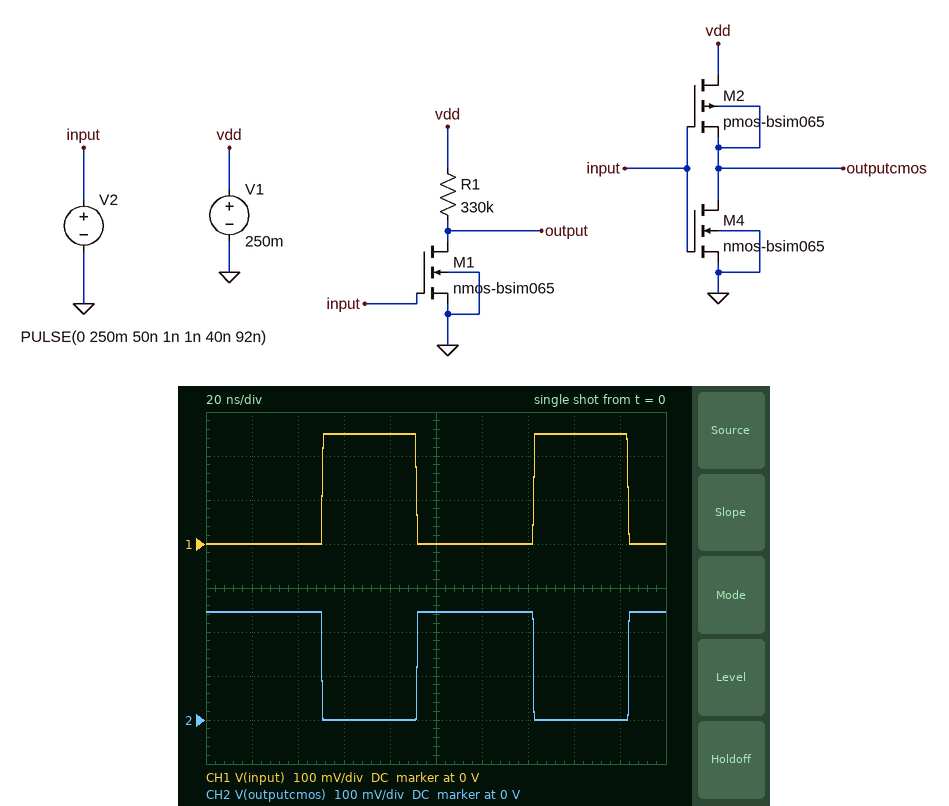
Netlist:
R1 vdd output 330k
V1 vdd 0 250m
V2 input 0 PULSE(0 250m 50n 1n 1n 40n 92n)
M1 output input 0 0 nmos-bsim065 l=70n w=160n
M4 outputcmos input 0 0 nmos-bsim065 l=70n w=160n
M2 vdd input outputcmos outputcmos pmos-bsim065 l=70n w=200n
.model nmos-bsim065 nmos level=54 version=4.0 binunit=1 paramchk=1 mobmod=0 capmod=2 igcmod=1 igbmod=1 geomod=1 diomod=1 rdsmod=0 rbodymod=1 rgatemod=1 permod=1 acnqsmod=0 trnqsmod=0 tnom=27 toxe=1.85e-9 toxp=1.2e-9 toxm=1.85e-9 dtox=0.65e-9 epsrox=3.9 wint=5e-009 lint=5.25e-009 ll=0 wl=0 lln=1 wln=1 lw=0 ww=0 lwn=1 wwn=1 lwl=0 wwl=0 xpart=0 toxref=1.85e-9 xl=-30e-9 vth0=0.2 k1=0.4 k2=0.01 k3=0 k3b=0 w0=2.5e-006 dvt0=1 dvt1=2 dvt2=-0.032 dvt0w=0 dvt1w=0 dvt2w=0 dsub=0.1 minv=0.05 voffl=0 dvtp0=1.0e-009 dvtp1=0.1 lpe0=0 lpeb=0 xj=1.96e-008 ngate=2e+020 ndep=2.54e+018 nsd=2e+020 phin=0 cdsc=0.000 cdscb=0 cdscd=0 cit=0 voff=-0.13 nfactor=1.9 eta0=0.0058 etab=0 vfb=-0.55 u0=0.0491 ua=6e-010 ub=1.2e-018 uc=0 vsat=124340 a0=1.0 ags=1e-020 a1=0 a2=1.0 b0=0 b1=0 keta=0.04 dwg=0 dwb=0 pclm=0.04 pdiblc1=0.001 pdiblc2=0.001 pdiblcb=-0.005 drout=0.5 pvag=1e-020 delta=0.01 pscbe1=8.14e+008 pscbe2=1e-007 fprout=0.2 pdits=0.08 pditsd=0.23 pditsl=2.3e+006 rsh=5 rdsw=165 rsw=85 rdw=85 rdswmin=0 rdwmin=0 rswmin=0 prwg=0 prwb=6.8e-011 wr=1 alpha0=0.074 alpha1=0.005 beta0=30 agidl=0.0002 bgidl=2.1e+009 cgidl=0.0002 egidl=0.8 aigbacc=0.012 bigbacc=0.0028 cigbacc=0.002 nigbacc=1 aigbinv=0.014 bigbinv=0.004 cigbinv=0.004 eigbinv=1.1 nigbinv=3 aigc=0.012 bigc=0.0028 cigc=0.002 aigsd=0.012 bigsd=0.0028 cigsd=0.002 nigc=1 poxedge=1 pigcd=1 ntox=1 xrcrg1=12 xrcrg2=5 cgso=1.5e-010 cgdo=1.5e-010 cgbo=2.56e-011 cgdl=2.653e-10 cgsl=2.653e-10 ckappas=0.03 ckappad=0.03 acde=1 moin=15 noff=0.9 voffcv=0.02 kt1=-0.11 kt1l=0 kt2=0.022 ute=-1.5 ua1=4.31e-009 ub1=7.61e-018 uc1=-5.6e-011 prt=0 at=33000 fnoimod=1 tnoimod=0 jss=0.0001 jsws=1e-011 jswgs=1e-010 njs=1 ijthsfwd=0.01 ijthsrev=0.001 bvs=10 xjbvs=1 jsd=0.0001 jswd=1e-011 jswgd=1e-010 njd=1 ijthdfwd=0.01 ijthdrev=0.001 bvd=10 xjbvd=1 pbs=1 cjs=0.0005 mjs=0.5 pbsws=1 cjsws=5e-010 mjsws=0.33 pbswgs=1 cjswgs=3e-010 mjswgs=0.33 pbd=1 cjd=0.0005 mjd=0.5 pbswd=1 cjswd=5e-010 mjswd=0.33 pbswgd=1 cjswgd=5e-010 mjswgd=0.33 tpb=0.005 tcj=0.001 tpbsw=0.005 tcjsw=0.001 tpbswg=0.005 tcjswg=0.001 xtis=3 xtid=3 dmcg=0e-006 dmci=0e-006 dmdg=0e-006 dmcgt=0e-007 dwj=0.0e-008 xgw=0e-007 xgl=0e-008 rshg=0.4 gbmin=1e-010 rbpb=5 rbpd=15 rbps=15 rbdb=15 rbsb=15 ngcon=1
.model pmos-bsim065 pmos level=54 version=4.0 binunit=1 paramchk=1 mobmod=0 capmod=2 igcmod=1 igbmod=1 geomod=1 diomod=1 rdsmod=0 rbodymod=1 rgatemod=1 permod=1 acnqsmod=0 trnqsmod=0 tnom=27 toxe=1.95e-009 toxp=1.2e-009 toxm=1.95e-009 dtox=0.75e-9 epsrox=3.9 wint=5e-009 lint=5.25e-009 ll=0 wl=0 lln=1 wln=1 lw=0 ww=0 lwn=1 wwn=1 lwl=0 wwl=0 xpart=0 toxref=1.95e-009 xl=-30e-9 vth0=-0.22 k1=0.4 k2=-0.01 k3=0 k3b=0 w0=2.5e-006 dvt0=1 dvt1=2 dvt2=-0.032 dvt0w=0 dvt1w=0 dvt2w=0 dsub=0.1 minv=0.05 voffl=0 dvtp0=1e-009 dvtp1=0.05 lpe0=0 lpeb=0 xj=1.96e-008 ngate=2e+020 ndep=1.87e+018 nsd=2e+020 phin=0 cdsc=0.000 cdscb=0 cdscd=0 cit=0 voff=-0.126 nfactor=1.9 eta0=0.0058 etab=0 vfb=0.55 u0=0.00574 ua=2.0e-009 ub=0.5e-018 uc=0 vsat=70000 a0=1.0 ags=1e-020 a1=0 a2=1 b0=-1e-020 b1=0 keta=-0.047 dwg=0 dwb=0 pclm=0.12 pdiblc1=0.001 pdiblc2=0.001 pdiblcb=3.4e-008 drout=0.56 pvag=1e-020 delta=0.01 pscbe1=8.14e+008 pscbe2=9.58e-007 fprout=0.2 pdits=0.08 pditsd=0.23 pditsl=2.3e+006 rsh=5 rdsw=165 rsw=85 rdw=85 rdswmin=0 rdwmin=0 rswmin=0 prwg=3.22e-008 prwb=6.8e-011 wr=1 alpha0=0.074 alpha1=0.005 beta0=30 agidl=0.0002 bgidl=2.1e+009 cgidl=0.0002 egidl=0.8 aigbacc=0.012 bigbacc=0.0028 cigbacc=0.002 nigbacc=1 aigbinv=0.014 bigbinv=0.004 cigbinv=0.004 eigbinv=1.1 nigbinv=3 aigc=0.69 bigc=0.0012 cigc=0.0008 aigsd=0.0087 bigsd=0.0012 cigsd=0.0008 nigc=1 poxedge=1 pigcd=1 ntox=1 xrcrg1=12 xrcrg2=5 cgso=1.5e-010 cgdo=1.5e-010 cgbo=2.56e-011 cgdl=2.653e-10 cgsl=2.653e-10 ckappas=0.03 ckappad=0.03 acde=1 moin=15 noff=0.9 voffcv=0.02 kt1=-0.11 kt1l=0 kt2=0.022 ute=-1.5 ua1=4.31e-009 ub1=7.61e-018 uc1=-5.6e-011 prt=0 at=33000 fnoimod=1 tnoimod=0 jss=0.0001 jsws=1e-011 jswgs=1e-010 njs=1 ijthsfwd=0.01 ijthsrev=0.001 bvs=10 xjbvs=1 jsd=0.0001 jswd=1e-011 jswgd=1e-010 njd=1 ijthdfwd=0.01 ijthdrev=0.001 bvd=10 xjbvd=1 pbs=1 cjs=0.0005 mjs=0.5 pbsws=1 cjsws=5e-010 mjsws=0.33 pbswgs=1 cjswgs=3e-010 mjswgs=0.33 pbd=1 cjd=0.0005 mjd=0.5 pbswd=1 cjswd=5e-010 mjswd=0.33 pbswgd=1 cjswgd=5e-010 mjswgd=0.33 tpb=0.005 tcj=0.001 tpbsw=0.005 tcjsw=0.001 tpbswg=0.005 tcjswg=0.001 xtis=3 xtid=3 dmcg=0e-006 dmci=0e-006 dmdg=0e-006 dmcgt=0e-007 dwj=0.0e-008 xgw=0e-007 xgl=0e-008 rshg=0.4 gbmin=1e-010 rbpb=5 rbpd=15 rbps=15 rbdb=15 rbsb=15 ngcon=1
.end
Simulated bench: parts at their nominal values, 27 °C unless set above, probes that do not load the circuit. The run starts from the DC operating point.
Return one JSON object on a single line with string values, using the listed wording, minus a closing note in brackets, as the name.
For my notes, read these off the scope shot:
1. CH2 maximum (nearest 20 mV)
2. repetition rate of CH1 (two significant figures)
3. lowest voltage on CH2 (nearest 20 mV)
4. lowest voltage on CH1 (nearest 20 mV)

{"CH2 maximum": "240 mV", "repetition rate of CH1": "11 MHz", "lowest voltage on CH2": "0 V", "lowest voltage on CH1": "0 V"}
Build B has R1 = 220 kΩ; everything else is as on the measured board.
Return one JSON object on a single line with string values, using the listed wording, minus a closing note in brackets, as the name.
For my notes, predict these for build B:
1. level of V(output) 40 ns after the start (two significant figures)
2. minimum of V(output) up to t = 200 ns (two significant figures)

{"level of V(output) 40 ns after the start": "230 mV", "minimum of V(output) up to t = 200 ns": "6.0 mV"}
